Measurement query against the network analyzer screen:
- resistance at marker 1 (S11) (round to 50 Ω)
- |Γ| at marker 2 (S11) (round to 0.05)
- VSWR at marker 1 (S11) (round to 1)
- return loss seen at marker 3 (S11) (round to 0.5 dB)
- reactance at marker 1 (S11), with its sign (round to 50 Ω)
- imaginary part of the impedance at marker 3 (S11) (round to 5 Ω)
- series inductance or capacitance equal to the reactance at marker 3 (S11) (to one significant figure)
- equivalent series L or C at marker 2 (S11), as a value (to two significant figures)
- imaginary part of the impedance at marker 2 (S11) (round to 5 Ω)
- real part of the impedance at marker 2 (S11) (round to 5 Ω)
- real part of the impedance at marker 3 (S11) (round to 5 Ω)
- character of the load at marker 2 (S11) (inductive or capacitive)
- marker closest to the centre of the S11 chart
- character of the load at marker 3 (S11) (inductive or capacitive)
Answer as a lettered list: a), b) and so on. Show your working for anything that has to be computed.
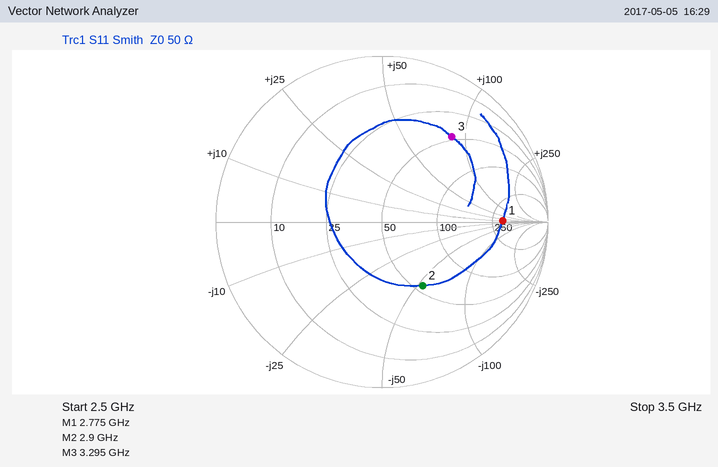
a) 300 Ω
b) 0.45
c) 6
d) 3.5 dB
e) 0 Ω
f) +85 Ω
g) L = 85 Ω/(2π × 3.295 GHz) ≈ 4 nH
h) C = 1/(2π × 2.9 GHz × 55 Ω) ≈ 1.0 pF
i) -55 Ω
j) 55 Ω
k) 45 Ω
l) capacitive
m) marker 2
n) inductive
